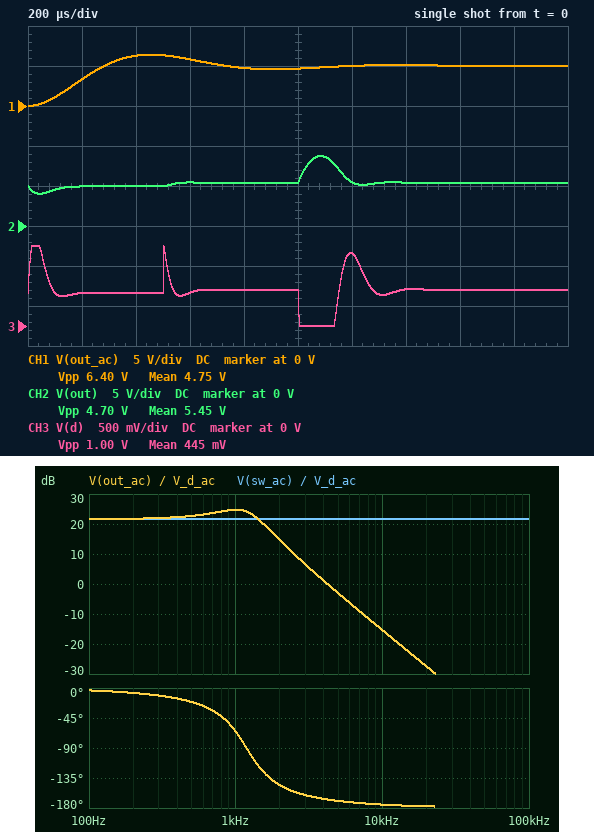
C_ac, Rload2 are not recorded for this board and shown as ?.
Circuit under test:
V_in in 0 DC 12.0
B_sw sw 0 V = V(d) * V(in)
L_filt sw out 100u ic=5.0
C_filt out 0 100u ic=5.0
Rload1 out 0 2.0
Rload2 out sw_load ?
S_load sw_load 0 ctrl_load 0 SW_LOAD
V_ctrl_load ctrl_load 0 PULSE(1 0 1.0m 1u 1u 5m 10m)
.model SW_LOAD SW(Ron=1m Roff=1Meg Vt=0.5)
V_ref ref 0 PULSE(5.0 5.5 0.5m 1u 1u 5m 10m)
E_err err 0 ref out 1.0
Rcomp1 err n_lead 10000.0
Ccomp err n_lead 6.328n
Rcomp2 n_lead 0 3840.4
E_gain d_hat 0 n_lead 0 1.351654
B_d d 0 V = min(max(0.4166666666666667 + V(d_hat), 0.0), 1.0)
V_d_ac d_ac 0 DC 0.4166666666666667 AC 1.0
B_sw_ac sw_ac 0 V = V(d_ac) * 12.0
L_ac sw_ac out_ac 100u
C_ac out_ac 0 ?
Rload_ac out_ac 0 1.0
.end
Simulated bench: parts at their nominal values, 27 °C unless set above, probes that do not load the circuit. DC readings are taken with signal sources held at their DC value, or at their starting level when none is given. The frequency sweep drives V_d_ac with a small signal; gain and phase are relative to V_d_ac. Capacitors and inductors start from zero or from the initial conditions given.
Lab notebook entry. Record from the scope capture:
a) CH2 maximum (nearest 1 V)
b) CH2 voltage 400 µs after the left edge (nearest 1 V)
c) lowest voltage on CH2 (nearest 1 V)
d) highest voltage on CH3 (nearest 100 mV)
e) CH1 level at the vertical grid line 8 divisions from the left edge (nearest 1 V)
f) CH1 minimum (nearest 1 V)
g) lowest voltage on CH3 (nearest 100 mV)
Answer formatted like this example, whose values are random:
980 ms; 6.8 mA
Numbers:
9 V; 5 V; 4 V; 1.0 V; 5 V; 0 V; 0 V
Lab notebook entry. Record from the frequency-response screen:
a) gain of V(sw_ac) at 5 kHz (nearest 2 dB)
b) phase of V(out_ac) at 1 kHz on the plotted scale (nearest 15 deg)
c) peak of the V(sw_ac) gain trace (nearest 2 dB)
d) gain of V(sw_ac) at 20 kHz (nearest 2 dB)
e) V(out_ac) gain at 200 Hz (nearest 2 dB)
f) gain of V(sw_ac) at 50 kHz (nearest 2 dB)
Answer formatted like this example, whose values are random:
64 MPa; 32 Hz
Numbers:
22 dB; -60 deg; 22 dB; 22 dB; 22 dB; 22 dB
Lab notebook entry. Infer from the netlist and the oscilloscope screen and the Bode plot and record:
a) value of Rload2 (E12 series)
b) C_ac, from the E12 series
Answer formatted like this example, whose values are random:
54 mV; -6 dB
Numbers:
0.68 Ω; 180 µF
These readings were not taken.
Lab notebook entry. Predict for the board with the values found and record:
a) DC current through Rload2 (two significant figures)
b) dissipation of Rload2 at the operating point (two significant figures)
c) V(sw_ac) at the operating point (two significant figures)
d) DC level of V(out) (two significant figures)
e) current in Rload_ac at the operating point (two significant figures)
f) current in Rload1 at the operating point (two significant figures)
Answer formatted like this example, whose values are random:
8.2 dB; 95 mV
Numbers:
7.3 A; 37 W; 5.0 V; 5.0 V; 5.0 A; 2.5 A
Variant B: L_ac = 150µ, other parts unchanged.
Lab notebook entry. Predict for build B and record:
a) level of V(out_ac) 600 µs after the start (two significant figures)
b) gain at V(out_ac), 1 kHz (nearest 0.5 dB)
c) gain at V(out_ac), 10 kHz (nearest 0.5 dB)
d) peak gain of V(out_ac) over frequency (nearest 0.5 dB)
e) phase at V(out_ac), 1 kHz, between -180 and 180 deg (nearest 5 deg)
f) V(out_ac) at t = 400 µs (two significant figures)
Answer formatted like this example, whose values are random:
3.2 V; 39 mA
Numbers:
6.0 V; 22.0 dB; -19.0 dB; 23.5 dB; -95 deg; 5.2 V
